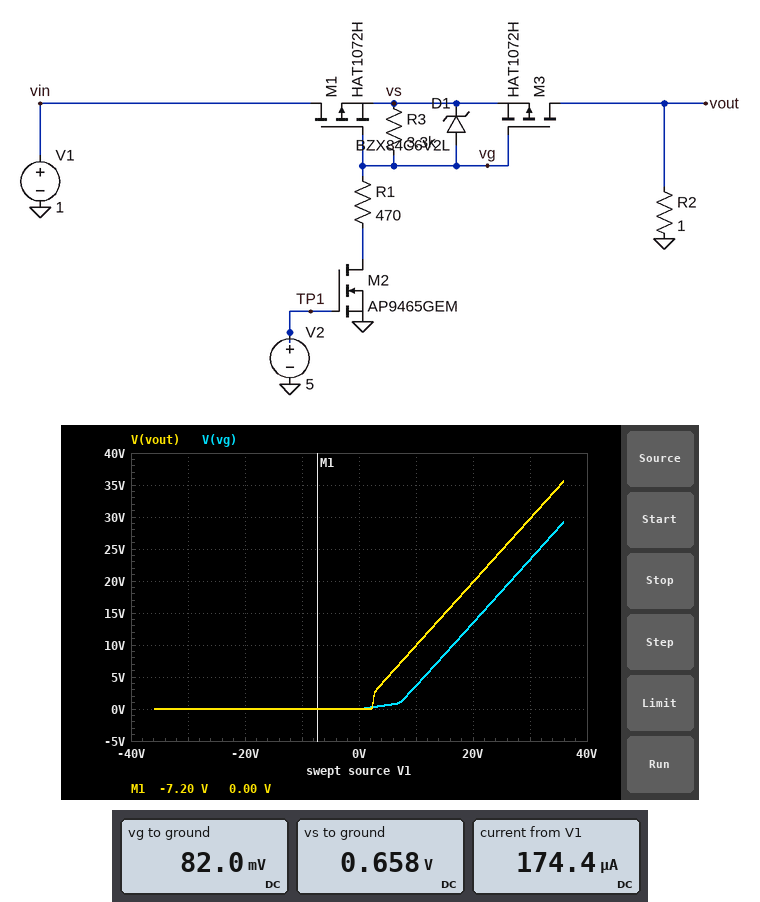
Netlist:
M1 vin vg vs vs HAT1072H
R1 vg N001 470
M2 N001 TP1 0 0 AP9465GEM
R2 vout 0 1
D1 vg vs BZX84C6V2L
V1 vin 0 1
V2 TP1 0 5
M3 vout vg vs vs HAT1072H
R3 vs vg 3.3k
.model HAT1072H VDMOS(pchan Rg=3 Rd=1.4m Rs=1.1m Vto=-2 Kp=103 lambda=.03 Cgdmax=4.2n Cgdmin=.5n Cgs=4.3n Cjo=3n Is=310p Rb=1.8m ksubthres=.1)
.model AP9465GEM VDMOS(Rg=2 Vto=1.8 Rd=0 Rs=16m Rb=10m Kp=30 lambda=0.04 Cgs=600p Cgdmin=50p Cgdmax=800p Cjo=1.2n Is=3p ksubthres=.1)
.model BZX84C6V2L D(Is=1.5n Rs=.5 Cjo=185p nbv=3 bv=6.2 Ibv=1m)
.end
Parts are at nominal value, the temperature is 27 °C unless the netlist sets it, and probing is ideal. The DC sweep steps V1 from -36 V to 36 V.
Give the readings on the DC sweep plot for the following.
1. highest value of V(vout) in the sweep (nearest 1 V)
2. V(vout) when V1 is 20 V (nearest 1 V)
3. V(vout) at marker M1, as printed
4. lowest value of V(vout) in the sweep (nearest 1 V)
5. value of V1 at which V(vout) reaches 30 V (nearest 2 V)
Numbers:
36 V
20 V
0.00 V
0 V
30 V
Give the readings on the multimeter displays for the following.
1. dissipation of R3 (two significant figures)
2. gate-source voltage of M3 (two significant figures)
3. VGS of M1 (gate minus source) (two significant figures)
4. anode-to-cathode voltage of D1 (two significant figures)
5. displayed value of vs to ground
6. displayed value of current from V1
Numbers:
100 µW
-580 mV
-580 mV
-580 mV
0.658 V
174.4 µA
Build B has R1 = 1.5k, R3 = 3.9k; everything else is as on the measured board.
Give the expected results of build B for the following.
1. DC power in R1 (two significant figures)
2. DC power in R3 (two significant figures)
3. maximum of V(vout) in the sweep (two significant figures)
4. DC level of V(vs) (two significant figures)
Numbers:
23 µW
59 µW
36 V
670 mV
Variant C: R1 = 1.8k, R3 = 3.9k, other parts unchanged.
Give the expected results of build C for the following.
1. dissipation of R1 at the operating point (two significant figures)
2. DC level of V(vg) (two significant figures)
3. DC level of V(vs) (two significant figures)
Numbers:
25 µW
210 mV
670 mV
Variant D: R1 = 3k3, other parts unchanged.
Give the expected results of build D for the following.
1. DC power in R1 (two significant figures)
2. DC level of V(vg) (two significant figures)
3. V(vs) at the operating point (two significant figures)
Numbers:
34 µW
340 mV
670 mV
